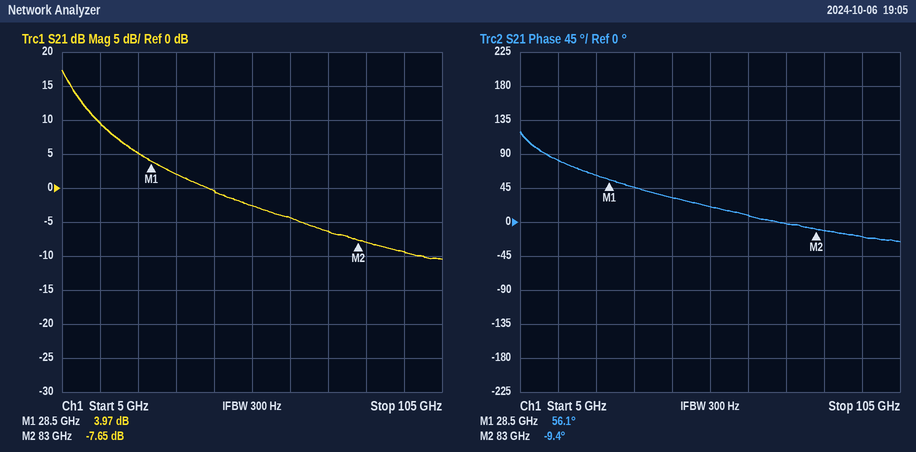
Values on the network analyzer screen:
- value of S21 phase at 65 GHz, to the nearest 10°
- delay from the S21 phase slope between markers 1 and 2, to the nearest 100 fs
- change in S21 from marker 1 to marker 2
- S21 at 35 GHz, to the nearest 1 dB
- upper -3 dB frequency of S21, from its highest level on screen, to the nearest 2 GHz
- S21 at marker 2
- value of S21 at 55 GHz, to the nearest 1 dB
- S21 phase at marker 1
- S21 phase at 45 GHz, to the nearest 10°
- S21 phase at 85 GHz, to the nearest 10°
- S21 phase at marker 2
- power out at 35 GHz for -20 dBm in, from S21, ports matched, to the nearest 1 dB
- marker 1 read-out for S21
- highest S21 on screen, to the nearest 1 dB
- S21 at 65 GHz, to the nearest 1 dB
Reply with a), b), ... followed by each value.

a) 10°
b) 3.3 ps
c) -11.62 dB
d) 2 dB
e) 8 GHz
f) -7.65 dB
g) -3 dB
h) 56.1°
i) 30°
j) -10°
k) -9.4°
l) -18 dBm
m) 3.97 dB
n) 17 dB
o) -4 dB
